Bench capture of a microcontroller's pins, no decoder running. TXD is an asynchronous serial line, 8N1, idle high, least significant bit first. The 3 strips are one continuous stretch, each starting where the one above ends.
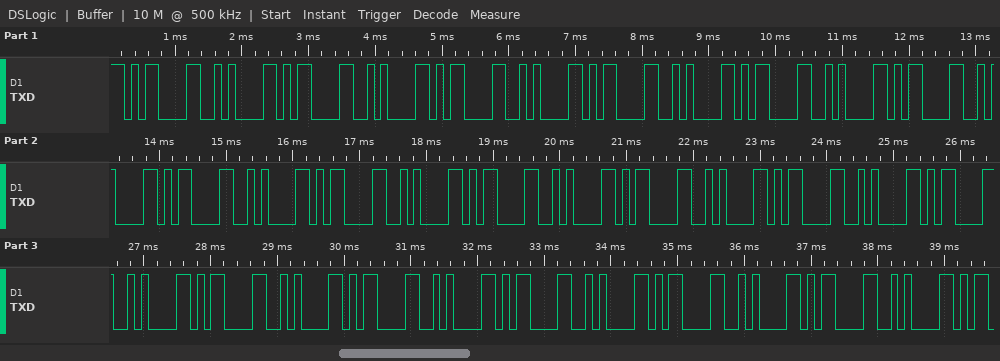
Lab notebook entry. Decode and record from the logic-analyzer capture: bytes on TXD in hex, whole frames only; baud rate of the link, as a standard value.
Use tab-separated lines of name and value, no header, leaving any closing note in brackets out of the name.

bytes on TXD in hex, whole frames only	0D 0A 0D 0A 0D 0A 0D 0A 0D 0A 0D 0A 0D 0A 0D 0A 0D 0A 0D 0A 0D 0A 0D 0A 0D 0A 0D 0A 0D 0A 0D 0A 0D 0A
baud rate of the link, as a standard value	9600 baud
